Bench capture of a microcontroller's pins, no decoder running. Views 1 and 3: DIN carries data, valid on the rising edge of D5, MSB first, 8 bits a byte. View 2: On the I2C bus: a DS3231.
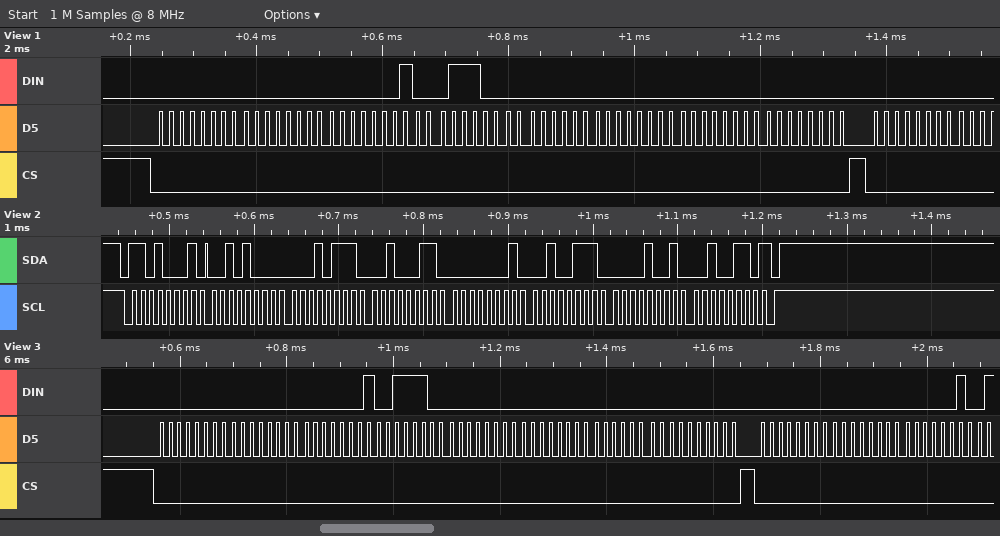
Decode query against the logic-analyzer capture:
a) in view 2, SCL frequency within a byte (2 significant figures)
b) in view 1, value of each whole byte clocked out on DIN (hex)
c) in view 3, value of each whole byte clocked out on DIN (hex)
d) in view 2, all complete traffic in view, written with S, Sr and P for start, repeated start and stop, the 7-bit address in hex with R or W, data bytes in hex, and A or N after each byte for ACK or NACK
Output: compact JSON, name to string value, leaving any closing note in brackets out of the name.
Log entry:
{"in view 2, SCL frequency within a byte": "100 kHz", "in view 1, value of each whole byte clocked out on DIN": "00 00 01 1C 00 00 00 00 00", "in view 3, value of each whole byte clocked out on DIN": "00 00 01 3C 00 00 00 00 00 00 02", "in view 2, all complete traffic in view, written with S, Sr and P for start, repeated start and stop, the 7-bit address in hex with R or W, data bytes in hex, and A or N after each byte for ACK or NACK": "S 68R A 28 A 17 A 23 A 01 A 27 A 09 A 26 N P"}
